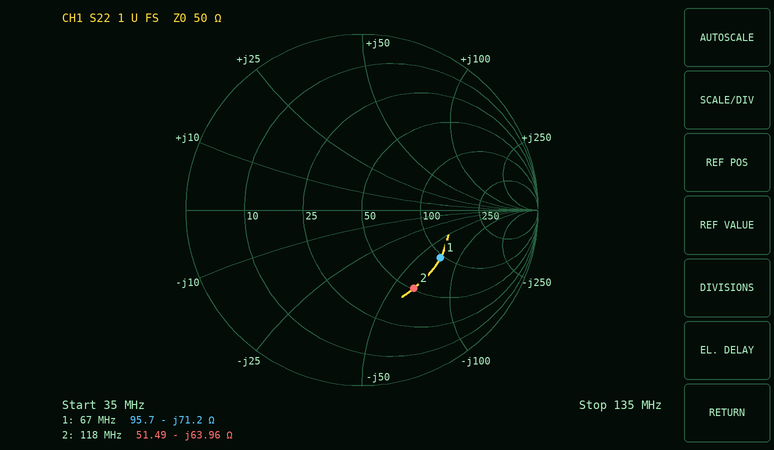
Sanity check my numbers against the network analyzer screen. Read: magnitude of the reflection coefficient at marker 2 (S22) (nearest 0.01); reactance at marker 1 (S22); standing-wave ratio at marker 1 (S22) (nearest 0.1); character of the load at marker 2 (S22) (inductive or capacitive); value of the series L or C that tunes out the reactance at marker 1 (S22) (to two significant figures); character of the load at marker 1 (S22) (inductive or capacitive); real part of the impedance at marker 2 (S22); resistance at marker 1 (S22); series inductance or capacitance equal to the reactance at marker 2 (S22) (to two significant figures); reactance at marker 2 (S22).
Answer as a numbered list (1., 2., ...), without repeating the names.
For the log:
1. 0.53
2. -71.2 Ω
3. 3.2
4. capacitive
5. 170 nH
6. capacitive
7. 51.49 Ω
8. 95.7 Ω
9. 21 pF
10. -63.96 Ω
